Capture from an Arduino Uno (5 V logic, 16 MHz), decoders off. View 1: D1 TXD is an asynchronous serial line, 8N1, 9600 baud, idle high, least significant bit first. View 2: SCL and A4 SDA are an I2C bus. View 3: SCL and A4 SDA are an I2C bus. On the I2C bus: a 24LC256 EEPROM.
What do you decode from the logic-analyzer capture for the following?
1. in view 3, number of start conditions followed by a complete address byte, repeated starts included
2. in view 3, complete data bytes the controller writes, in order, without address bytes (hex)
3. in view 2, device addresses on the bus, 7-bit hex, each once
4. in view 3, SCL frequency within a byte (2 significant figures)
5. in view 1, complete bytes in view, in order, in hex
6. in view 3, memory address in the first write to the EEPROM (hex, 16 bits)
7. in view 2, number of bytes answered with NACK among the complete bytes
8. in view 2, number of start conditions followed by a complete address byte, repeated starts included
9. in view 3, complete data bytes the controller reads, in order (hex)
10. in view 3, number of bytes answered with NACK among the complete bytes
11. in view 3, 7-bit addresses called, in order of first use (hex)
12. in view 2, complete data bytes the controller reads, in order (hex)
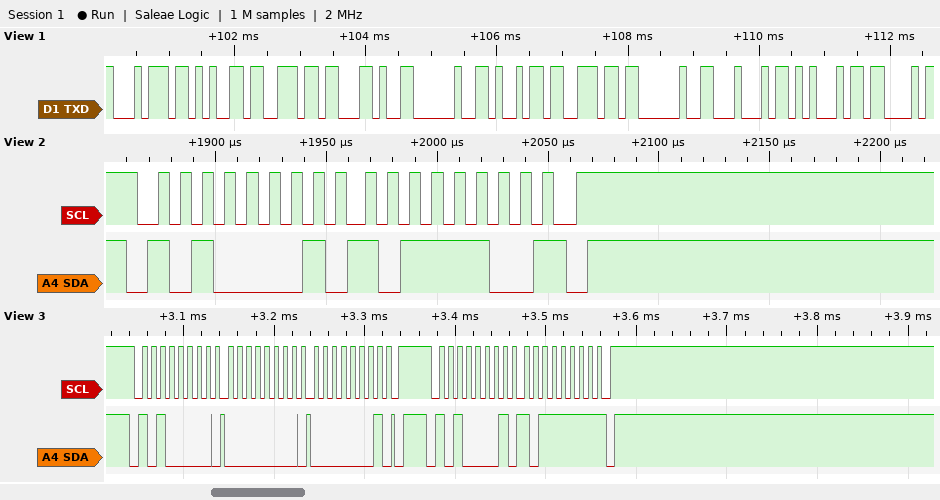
2
00 01
0x50
100 kHz
74 65 6E 2C 20 69 6E 20 44 45 43
0x0001
1
1
BF
1
0x50
BC
